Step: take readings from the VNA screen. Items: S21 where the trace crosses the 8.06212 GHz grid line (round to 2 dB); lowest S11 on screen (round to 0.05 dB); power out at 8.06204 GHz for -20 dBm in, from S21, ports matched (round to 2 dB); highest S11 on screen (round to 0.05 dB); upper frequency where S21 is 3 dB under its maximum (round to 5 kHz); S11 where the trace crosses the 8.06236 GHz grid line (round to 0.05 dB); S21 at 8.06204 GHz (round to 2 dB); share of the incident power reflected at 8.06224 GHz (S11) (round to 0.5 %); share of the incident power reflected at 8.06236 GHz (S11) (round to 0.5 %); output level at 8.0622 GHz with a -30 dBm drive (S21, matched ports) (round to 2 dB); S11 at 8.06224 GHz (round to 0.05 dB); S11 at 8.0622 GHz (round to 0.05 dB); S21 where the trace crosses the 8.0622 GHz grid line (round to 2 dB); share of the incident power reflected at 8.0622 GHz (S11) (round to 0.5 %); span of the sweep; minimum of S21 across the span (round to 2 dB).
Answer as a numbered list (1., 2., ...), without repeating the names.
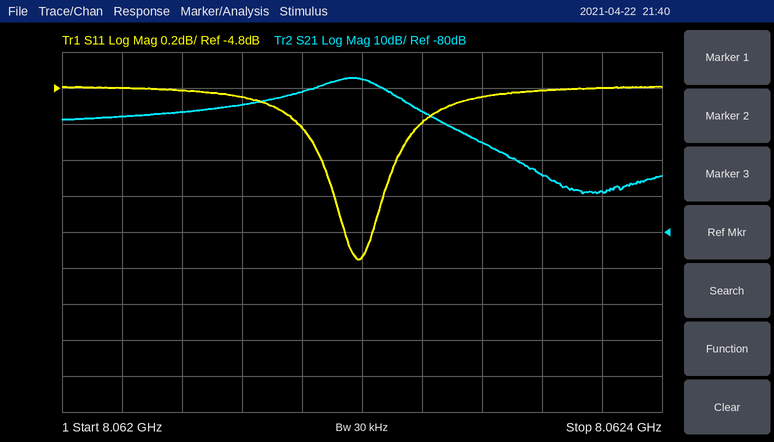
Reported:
1. -44 dB
2. -5.75 dB
3. -68 dBm
4. -4.80 dB
5. 8.062215 GHz
6. -4.80 dB
7. -48 dB
8. 31.5 %
9. 33.0 %
10. -68 dBm
11. -5.00 dB
12. -5.75 dB
13. -38 dB
14. 26.5 %
15. 400 kHz
16. -70 dB
